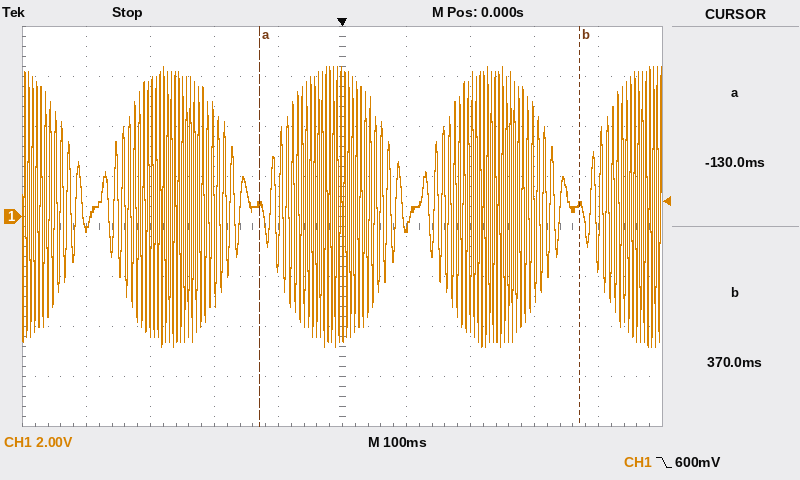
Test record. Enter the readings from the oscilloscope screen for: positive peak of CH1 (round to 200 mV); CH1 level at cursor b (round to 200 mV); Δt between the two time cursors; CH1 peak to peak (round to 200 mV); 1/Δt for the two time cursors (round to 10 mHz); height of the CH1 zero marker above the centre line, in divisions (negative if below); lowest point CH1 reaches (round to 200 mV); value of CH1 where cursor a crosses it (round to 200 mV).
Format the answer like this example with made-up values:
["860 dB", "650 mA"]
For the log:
["6.0 V", "400 mV", "500 ms", "11.2 V", "2.00 Hz", "+0.2 div", "-5.2 V", "400 mV"]
